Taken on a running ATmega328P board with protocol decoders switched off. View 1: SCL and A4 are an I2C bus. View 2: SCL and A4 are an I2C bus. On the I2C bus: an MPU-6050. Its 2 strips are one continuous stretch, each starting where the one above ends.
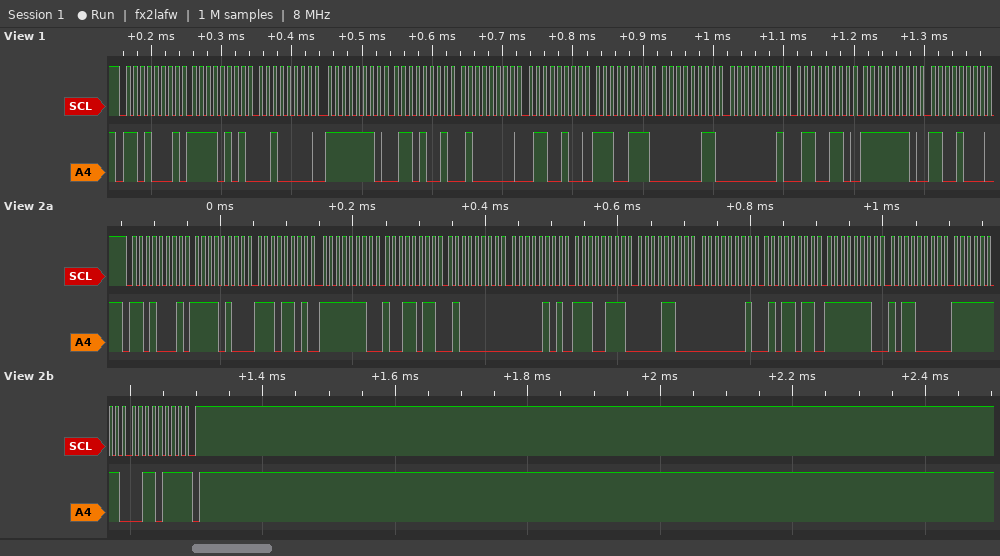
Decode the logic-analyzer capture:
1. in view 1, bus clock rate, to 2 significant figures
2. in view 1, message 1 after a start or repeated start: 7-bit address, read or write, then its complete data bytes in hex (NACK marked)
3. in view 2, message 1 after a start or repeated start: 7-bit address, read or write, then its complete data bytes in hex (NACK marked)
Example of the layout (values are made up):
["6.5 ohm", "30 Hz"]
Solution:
["100 kHz", "0x68 read: F5 20 FE 69 40 64 E7 03 01 66 FE C8", "0x68 read: F4 ED FE 9B 40 05 E7 0C 01 5B FE B0 FF 37 NACK"]
